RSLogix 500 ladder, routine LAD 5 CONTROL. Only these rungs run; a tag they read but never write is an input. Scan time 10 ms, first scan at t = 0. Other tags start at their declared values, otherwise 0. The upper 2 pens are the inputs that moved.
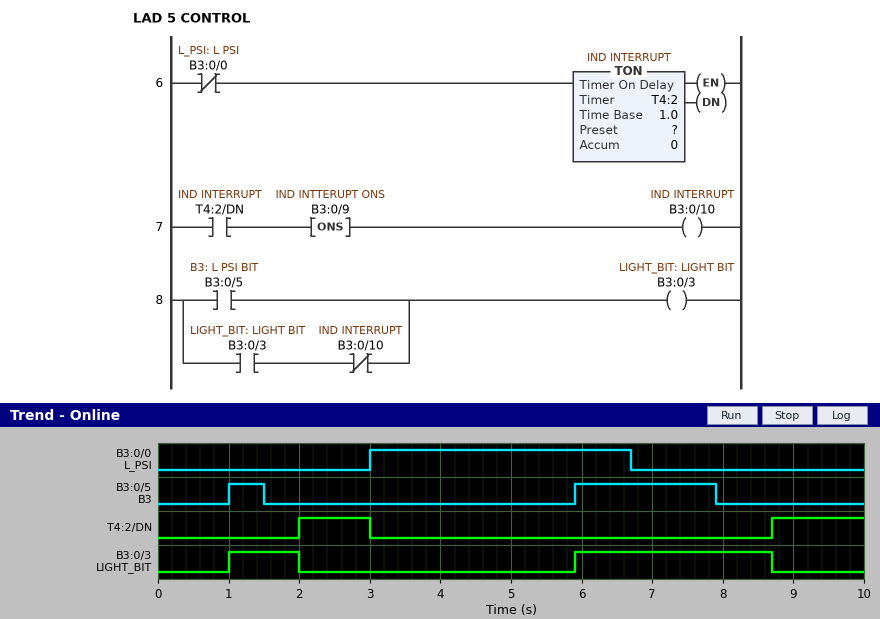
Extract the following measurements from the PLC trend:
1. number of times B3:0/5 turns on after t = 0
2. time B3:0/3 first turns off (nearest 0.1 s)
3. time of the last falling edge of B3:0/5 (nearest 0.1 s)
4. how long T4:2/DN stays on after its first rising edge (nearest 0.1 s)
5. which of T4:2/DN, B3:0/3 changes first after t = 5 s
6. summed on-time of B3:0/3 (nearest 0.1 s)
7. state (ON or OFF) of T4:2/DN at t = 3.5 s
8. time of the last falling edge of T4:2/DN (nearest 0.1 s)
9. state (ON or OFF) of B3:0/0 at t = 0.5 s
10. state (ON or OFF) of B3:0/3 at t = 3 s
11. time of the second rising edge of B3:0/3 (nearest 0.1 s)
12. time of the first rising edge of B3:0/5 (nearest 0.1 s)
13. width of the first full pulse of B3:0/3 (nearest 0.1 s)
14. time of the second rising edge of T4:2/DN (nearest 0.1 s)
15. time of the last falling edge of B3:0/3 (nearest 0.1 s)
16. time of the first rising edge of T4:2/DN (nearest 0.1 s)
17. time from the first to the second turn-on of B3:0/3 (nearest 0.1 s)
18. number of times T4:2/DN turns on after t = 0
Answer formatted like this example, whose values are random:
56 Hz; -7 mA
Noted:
2; 2.0 s; 7.9 s; 1.0 s; B3:0/3; 3.8 s; OFF; 3.0 s; OFF; OFF; 5.9 s; 1.0 s; 1.0 s; 8.7 s; 8.7 s; 2.0 s; 4.9 s; 2
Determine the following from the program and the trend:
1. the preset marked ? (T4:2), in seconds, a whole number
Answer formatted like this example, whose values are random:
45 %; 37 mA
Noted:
2 s
